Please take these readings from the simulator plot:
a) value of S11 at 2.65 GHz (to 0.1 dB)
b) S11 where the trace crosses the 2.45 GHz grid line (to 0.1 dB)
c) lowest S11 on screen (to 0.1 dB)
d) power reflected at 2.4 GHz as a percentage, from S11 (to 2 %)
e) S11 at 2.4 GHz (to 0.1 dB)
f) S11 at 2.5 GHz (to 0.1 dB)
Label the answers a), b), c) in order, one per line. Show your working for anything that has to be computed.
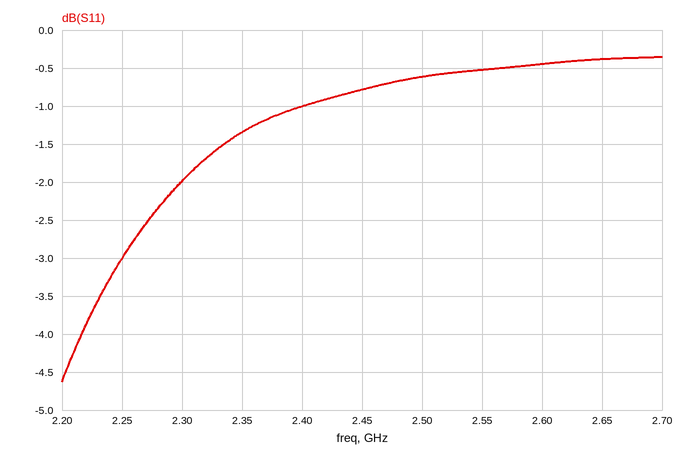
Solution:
a) -0.4 dB
b) -0.8 dB
c) -4.6 dB
d) 10^(-1/10) ≈ 79.4 %, so 80 % to the nearest 2 %
e) -1.0 dB
f) -0.6 dB
